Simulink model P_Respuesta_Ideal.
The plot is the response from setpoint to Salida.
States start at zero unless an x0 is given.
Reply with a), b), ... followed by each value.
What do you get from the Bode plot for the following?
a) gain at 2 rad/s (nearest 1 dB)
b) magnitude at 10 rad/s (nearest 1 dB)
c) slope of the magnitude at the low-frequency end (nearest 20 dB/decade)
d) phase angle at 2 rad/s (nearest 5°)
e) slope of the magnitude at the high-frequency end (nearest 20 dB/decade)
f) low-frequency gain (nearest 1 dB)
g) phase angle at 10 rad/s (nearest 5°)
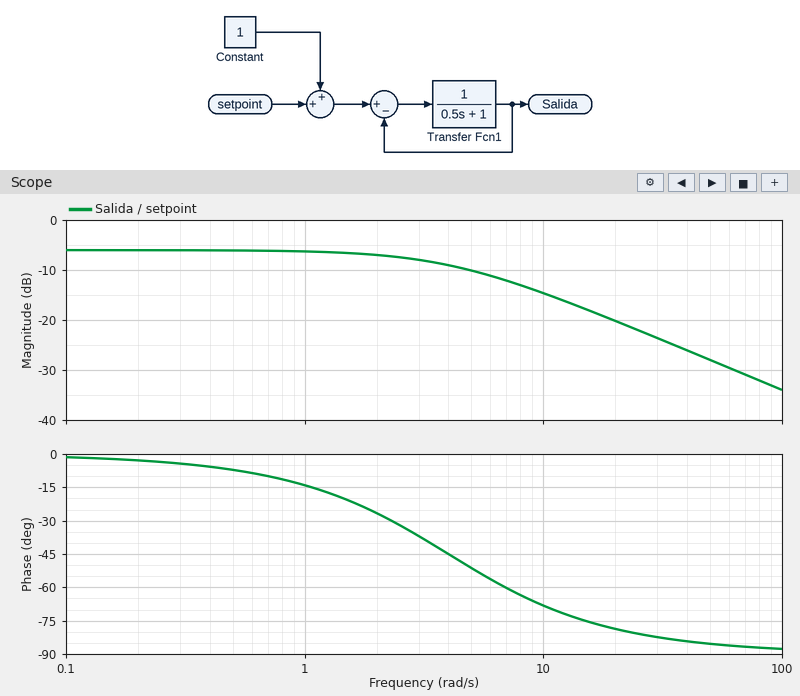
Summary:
a) -7 dB
b) -15 dB
c) 0 dB/decade
d) -25°
e) -20 dB/decade
f) -6 dB
g) -70°
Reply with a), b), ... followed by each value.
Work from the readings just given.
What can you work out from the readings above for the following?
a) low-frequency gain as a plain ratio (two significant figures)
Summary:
a) 0.50
